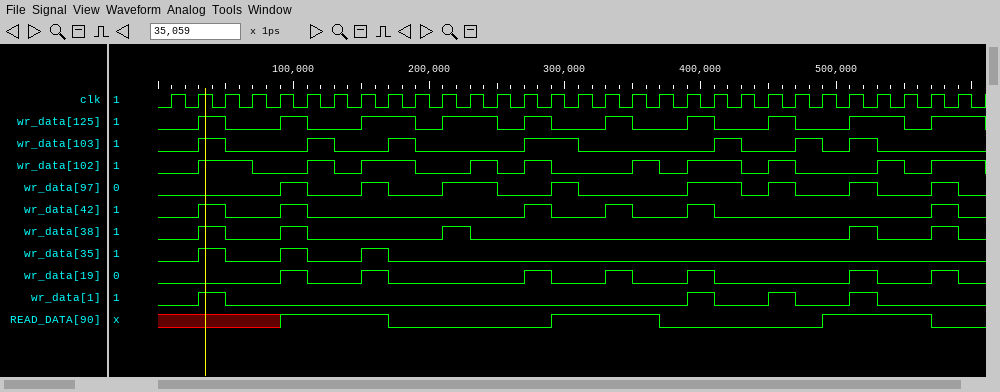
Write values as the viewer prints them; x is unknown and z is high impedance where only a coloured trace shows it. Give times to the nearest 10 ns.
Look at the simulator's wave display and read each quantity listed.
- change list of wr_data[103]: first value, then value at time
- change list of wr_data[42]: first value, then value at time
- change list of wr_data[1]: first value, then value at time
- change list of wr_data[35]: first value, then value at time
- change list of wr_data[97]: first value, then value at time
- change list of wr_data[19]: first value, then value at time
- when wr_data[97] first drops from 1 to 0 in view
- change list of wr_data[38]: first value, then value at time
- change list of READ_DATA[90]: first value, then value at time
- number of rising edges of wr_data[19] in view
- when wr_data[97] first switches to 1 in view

0, 1 at 30 ns, 0 at 50 ns, 1 at 110 ns, 0 at 130 ns, 1 at 170 ns, 0 at 190 ns, 1 at 270 ns, 0 at 310 ns, 1 at 410 ns, 0 at 430 ns, 1 at 470 ns, 0 at 490 ns, 1 at 510 ns, 0 at 530 ns
0, 1 at 30 ns, 0 at 50 ns, 1 at 90 ns, 0 at 110 ns, 1 at 270 ns, 0 at 290 ns, 1 at 330 ns, 0 at 350 ns, 1 at 390 ns, 0 at 410 ns, 1 at 570 ns, 0 at 590 ns
0, 1 at 30 ns, 0 at 50 ns, 1 at 390 ns, 0 at 410 ns, 1 at 450 ns, 0 at 470 ns, 1 at 510 ns, 0 at 530 ns
0, 1 at 30 ns, 0 at 50 ns, 1 at 90 ns, 0 at 110 ns, 1 at 150 ns, 0 at 170 ns
0, 1 at 90 ns, 0 at 110 ns, 1 at 150 ns, 0 at 170 ns, 1 at 210 ns, 0 at 250 ns, 1 at 290 ns, 0 at 310 ns, 1 at 390 ns, 0 at 430 ns, 1 at 450 ns, 0 at 470 ns, 1 at 510 ns, 0 at 530 ns, 1 at 570 ns, 0 at 590 ns
0, 1 at 90 ns, 0 at 110 ns, 1 at 150 ns, 0 at 170 ns, 1 at 270 ns, 0 at 290 ns, 1 at 330 ns, 0 at 350 ns, 1 at 390 ns, 0 at 410 ns, 1 at 510 ns, 0 at 530 ns, 1 at 570 ns, 0 at 590 ns
110 ns
0, 1 at 30 ns, 0 at 50 ns, 1 at 90 ns, 0 at 110 ns, 1 at 210 ns, 0 at 230 ns, 1 at 510 ns, 0 at 530 ns, 1 at 570 ns, 0 at 590 ns
x, 1 at 90 ns, 0 at 170 ns, 1 at 290 ns, 0 at 370 ns, 1 at 490 ns, 0 at 570 ns
7
90 ns
